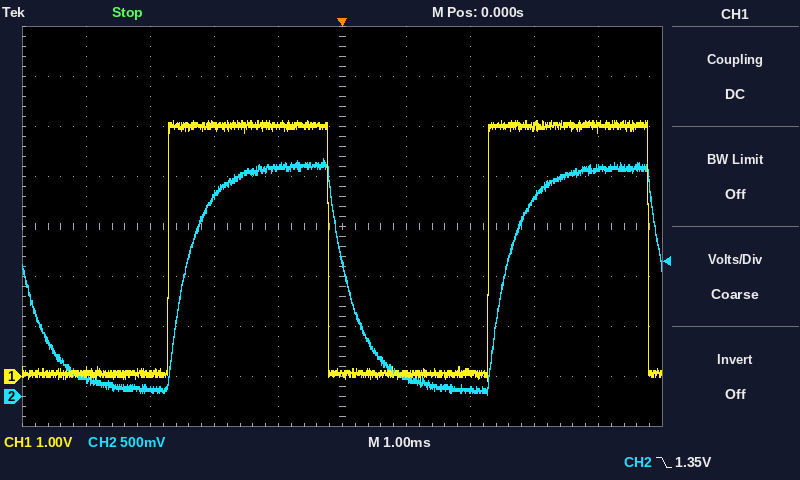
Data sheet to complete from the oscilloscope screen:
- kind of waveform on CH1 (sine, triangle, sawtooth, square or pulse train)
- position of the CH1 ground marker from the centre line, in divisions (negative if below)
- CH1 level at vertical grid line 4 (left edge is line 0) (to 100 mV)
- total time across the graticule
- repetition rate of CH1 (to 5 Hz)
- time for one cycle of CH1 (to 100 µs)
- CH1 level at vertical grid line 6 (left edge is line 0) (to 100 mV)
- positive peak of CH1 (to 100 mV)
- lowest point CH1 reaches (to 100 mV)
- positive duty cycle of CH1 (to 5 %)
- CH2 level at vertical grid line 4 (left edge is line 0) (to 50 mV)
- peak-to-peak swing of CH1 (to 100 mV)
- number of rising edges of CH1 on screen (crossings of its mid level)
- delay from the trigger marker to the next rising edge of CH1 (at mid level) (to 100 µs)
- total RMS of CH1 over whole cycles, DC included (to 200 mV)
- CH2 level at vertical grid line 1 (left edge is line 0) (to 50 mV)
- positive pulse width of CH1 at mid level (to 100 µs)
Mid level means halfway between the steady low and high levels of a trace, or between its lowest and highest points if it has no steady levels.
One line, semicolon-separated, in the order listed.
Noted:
square; -3.0 div; 5.0 V; 10 ms; 200 Hz; 5.0 ms; 100 mV; 5.1 V; -100 mV; 50 %; 2.30 V; 5.2 V; 2; 2.3 ms; 3.6 V; 150 mV; 2.5 ms
